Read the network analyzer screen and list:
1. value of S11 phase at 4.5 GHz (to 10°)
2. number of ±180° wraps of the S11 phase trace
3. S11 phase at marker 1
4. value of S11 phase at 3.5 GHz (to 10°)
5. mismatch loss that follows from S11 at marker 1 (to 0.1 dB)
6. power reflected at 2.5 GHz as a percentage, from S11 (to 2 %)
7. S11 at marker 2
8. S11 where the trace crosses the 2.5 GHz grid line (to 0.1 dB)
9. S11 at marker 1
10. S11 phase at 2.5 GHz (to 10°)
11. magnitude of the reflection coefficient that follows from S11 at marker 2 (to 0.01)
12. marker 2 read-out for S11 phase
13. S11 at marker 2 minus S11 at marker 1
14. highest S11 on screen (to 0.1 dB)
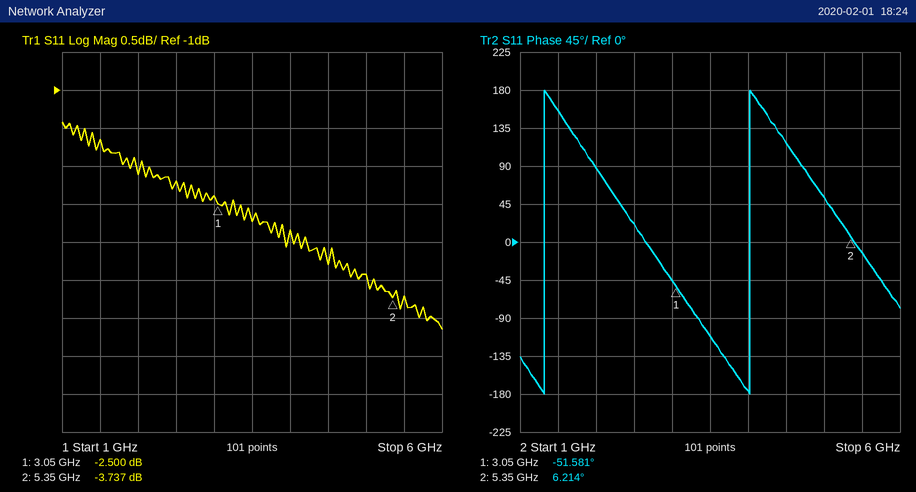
120°
2
-51.581°
-110°
3.6 dB
60 %
-3.737 dB
-2.2 dB
-2.500 dB
20°
0.65
6.214°
-1.237 dB
-1.4 dB
